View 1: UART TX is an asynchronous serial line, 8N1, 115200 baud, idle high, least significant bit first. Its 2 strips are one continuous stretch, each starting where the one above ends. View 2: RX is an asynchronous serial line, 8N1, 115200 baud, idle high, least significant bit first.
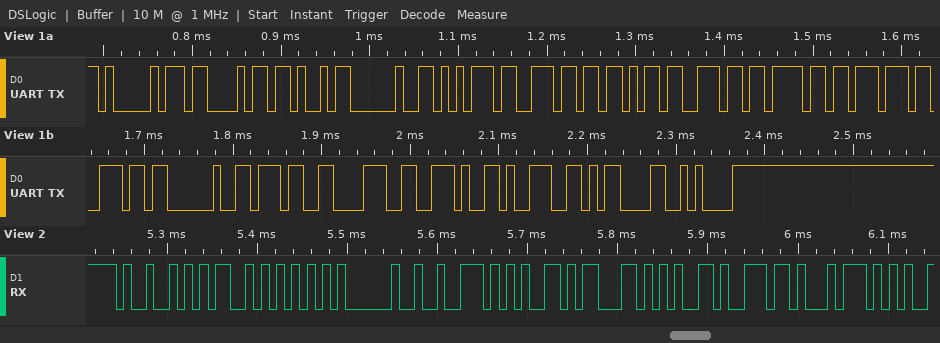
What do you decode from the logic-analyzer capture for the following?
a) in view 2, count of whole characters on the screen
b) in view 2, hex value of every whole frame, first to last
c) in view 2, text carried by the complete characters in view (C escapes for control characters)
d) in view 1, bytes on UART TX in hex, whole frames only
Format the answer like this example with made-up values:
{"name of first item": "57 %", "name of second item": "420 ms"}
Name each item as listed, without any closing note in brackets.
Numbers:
{"in view 2, count of whole characters on the screen": "10", "in view 2, hex value of every whole frame, first to last": "49 4D 55 20 72 65 63 65 6E 74", "in view 2, text carried by the complete characters in view": "\"IMU recent\"", "in view 1, bytes on UART TX in hex, whole frames only": "41 43 4B 20 75 6E 6B 6E 6F 77 6E 20 37 38 2E 39 0D 0A"}
